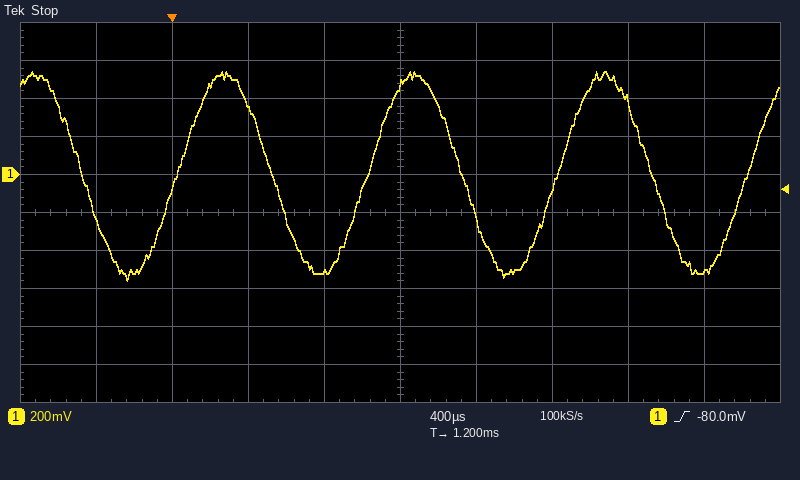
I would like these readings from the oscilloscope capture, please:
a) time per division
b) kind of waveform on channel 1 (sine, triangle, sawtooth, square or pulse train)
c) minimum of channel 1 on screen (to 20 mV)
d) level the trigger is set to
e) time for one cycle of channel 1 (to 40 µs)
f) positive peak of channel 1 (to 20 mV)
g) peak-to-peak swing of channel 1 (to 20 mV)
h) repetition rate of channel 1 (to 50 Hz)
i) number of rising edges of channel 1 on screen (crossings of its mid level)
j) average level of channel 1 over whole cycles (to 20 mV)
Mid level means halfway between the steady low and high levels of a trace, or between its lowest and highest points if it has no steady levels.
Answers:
400 µs
sine
-560 mV
-80.0 mV
1.00 ms
540 mV
1.10 V
1.00 kHz
4
0 mV
